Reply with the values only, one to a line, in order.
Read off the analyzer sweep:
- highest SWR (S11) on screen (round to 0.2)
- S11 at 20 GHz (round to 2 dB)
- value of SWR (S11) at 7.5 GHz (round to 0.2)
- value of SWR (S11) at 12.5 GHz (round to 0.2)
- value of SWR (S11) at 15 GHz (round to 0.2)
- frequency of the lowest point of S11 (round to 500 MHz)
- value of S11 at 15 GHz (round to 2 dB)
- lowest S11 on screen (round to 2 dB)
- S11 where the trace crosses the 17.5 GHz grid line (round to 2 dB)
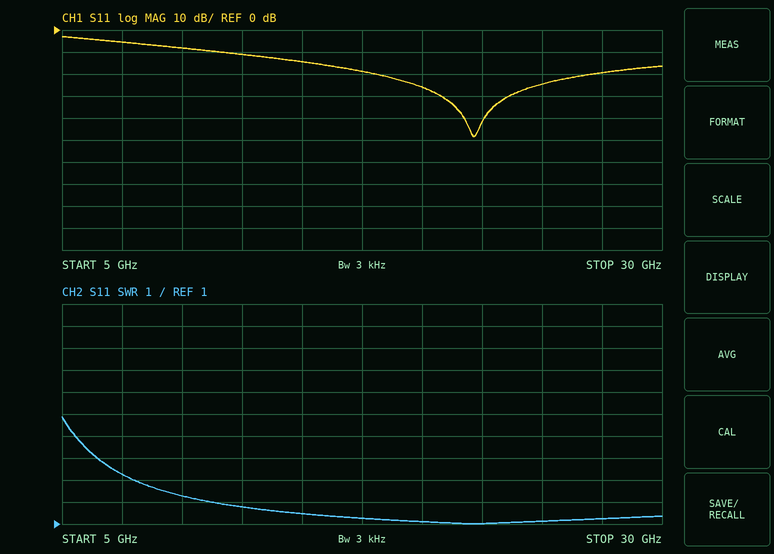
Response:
5.8
-26 dB
3.2
1.8
1.4
22.0 GHz
-14 dB
-48 dB
-18 dB
